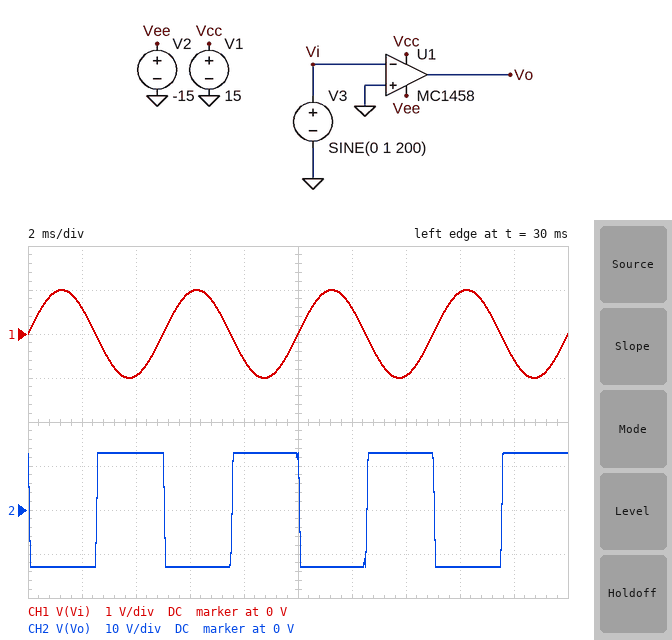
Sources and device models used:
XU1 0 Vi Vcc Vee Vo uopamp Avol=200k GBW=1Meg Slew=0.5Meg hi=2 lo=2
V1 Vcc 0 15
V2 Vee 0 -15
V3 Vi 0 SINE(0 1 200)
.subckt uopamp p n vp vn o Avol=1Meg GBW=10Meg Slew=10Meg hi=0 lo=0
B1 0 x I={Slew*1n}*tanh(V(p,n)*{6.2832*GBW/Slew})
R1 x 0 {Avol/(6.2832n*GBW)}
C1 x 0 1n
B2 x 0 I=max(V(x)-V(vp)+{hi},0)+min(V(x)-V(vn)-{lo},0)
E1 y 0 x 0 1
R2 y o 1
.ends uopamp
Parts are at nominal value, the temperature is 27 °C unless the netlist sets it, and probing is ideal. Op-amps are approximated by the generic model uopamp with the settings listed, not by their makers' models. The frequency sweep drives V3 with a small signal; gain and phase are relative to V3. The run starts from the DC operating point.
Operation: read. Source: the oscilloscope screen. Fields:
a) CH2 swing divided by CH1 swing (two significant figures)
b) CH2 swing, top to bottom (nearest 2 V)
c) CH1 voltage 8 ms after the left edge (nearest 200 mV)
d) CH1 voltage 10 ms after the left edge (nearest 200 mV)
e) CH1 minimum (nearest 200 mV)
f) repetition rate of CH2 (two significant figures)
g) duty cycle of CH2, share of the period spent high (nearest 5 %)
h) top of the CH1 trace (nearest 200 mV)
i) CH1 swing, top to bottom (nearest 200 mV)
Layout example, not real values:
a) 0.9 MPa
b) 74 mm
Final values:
a) 13
b) 26 V
c) -600 mV
d) 0 V
e) -1.0 V
f) 200 Hz
g) 50 %
h) 1.0 V
i) 2.0 V
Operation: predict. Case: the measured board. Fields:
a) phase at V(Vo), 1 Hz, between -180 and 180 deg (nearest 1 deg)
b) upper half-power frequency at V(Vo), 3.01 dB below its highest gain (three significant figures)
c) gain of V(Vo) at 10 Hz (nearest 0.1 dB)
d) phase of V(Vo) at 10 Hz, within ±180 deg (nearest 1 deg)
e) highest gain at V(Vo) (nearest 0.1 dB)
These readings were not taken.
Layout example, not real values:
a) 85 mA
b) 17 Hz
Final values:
a) 169 deg
b) 5.00 Hz
c) 99.0 dB
d) 117 deg
e) 106.0 dB
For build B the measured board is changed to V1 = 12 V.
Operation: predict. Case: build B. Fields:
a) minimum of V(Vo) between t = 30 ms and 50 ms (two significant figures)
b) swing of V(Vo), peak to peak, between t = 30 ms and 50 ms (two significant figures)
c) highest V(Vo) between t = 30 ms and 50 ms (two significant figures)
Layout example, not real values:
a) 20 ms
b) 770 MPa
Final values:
a) -13 V
b) 23 V
c) 10 V
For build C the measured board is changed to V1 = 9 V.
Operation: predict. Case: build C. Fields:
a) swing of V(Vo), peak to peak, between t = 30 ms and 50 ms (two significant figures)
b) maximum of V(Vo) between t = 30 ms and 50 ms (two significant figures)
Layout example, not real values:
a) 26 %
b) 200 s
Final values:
a) 20 V
b) 7.0 V
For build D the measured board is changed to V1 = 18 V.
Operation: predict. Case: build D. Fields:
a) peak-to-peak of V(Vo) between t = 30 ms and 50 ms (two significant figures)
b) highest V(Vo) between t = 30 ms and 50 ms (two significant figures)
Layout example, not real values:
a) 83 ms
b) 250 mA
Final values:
a) 29 V
b) 16 V
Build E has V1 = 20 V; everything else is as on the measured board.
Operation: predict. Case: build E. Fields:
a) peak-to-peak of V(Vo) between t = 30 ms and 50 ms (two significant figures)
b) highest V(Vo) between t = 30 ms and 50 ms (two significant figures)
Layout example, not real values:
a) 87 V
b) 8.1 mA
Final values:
a) 31 V
b) 18 V
